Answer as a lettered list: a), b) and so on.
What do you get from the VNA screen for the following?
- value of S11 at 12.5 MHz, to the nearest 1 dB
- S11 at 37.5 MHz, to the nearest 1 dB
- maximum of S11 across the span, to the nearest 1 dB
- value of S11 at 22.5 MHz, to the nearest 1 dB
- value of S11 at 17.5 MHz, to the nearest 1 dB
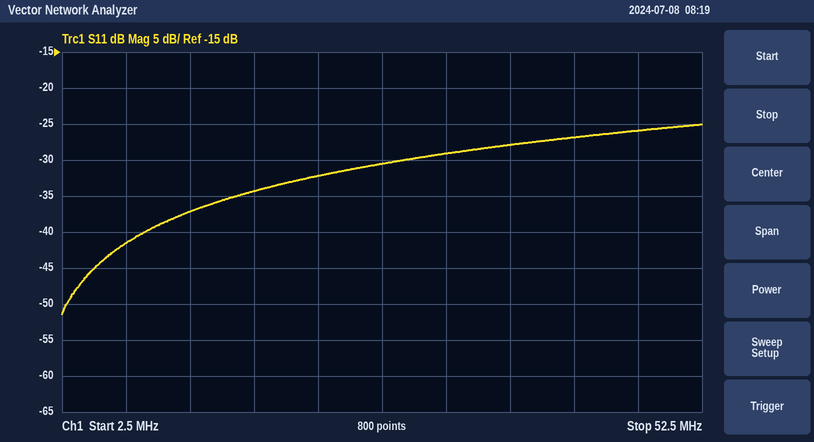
a) -37 dB
b) -28 dB
c) -25 dB
d) -32 dB
e) -34 dB
